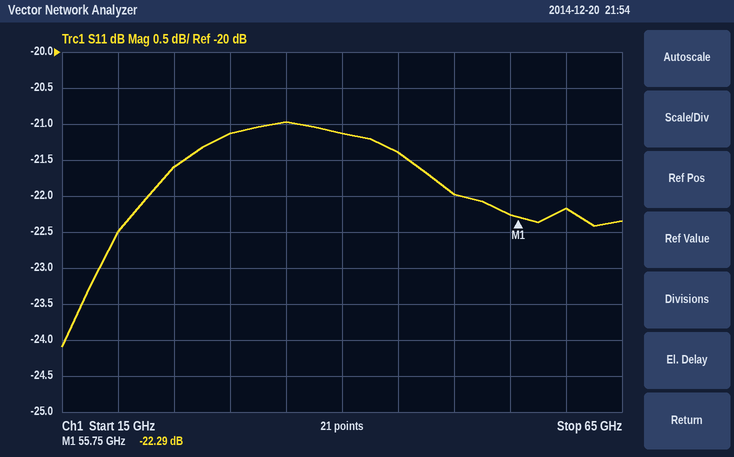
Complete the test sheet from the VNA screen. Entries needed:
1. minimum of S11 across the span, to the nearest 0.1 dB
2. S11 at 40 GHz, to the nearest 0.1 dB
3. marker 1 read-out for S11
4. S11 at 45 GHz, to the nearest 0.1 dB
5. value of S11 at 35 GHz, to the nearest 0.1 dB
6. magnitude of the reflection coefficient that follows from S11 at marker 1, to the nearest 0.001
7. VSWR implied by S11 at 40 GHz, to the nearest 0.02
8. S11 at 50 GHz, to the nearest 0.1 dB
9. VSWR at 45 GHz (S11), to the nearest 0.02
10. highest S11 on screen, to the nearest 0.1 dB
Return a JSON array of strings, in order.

["-24.1 dB", "-21.1 dB", "-22.29 dB", "-21.4 dB", "-21.0 dB", "0.077", "1.20", "-22.0 dB", "1.18", "-21.0 dB"]
